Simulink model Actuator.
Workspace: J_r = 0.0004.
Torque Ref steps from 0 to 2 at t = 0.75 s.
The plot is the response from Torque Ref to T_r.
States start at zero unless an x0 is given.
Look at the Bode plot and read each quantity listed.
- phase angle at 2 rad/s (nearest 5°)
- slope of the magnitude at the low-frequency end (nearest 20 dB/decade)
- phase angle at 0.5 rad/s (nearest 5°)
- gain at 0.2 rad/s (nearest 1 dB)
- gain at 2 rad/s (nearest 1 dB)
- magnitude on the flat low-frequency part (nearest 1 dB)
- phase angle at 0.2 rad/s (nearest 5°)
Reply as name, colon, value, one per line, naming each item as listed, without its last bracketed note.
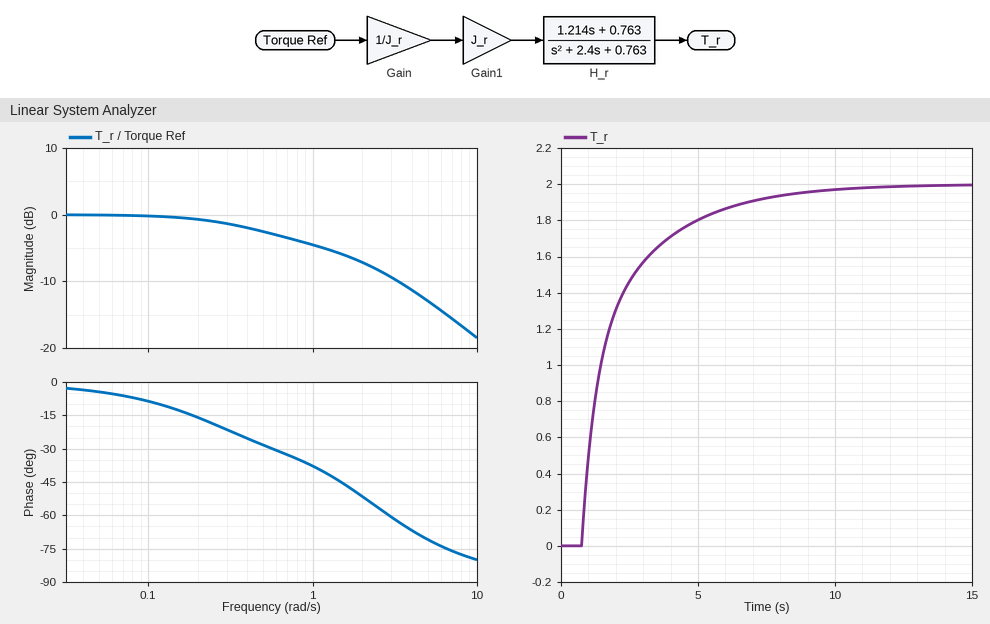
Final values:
phase angle at 2 rad/s: -50°
slope of the magnitude at the low-frequency end: 0 dB/decade
phase angle at 0.5 rad/s: -30°
gain at 0.2 rad/s: -1 dB
gain at 2 rad/s: -7 dB
magnitude on the flat low-frequency part: 0 dB
phase angle at 0.2 rad/s: -15°
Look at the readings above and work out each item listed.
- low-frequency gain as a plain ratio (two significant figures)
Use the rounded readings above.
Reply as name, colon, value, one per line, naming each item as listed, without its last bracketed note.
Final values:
low-frequency gain as a plain ratio: 1.0
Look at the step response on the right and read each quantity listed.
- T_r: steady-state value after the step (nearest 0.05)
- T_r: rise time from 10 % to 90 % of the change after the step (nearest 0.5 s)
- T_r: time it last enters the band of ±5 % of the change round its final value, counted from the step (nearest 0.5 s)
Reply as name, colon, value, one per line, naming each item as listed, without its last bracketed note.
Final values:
T_r: steady-state value after the step: 2.00
T_r: rise time from 10 % to 90 % of the change after the step: 4.0 s
T_r: time it last enters the band of ±5 % of the change round its final value, counted from the step: 6.0 s
